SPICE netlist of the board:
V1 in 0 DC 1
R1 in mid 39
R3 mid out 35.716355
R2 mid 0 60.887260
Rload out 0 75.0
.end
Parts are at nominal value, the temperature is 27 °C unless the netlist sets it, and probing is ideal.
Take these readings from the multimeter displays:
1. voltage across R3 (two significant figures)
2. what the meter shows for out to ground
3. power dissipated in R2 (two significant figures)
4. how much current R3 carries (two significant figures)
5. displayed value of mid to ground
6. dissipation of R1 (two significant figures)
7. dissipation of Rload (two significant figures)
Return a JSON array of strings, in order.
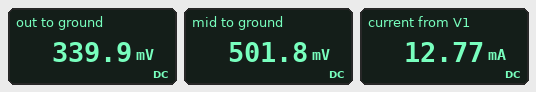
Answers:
["160 mV", "339.9 mV", "4.1 mW", "4.5 mA", "501.8 mV", "6.4 mW", "1.5 mW"]
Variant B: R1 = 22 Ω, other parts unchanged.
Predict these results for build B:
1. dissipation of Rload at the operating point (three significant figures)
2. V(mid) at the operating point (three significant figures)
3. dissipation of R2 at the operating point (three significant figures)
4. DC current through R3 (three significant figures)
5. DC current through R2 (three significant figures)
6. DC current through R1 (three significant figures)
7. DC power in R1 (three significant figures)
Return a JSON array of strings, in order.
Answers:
["2.51 mW", "641 mV", "6.75 mW", "5.79 mA", "10.5 mA", "16.3 mA", "5.86 mW"]
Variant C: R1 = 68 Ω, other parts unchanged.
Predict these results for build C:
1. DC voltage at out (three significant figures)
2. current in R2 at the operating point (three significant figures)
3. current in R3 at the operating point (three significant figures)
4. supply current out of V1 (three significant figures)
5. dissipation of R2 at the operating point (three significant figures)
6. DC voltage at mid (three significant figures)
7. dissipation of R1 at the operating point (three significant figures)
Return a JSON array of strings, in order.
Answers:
["248 mV", "6.01 mA", "3.31 mA", "9.32 mA", "2.20 mW", "366 mV", "5.91 mW"]
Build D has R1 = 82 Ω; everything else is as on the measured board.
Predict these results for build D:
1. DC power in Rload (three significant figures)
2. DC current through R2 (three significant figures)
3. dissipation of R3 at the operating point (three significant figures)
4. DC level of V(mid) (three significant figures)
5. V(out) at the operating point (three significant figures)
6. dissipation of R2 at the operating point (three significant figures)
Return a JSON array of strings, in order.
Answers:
["642 µW", "5.32 mA", "306 µW", "324 mV", "219 mV", "1.72 mW"]
